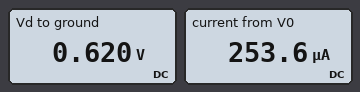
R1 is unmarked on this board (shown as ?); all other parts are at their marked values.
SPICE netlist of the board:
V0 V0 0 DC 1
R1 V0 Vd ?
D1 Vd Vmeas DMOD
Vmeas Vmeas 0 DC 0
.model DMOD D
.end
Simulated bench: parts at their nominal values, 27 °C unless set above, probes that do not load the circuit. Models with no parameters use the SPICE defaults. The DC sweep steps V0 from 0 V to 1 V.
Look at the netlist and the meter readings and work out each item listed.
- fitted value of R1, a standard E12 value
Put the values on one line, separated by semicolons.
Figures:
1.5 kΩ
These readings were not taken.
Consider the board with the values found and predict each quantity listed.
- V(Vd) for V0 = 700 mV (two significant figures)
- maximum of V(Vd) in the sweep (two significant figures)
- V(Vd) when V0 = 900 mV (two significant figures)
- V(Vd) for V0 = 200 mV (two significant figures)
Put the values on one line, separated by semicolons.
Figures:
590 mV; 620 mV; 610 mV; 200 mV
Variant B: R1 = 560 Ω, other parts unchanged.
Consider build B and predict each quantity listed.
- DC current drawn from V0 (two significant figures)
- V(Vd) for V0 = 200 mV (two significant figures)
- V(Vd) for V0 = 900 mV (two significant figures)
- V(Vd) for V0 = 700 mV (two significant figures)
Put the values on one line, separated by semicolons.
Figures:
640 µA; 200 mV; 640 mV; 610 mV
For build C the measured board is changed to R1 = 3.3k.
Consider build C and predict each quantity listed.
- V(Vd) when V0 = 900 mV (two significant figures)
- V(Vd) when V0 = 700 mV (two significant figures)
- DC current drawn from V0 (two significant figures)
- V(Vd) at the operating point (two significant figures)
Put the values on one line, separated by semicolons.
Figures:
590 mV; 570 mV; 120 µA; 600 mV
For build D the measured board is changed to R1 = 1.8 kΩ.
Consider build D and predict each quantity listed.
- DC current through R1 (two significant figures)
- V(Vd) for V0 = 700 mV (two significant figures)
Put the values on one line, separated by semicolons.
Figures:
210 µA; 580 mV
